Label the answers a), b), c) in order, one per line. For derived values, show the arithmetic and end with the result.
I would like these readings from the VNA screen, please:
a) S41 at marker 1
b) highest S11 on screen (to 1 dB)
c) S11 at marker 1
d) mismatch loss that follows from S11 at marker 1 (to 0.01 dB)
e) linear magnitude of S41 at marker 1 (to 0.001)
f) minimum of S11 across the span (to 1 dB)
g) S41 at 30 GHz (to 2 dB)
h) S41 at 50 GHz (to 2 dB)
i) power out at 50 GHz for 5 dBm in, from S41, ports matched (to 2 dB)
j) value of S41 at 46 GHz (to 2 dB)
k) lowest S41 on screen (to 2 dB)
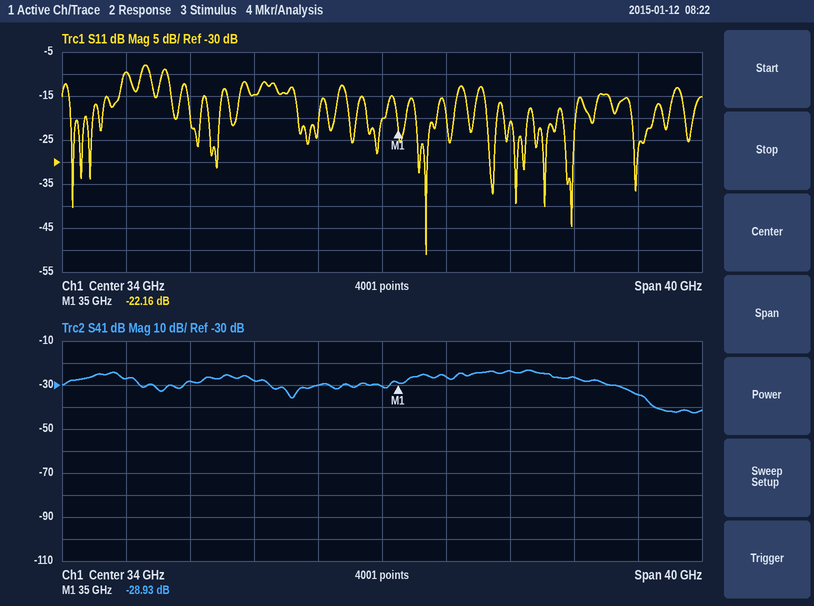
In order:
a) -28.93 dB
b) -8 dB
c) -22.16 dB
d) −10 log10(1 − 10^(-22.16/10)) ≈ 0.03 dB
e) 10^(-28.93/20) ≈ 0.036
f) -51 dB
g) -30 dB
h) -34 dB
i) 5 dBm + (-34 dB) = -30 dBm
j) -26 dB
k) -42 dB
